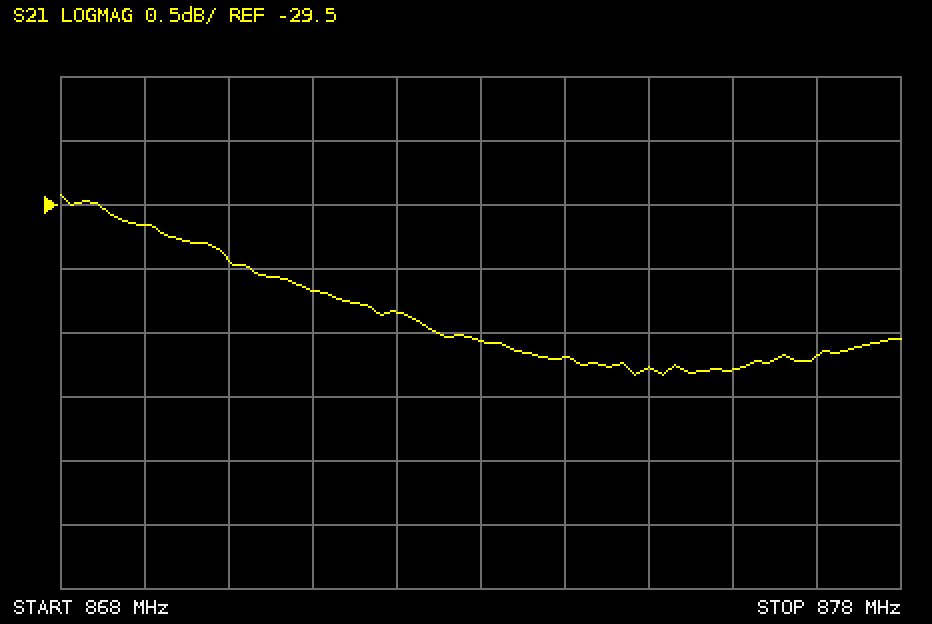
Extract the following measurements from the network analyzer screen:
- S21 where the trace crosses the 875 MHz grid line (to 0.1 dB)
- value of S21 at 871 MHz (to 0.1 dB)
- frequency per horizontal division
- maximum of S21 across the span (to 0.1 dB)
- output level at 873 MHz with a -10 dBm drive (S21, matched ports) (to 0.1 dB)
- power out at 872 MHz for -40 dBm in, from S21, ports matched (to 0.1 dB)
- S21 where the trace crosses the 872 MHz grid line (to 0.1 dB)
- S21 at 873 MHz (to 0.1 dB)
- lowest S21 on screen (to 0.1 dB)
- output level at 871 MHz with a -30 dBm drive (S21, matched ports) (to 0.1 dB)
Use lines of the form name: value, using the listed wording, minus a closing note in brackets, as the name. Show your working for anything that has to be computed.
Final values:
S21 where the trace crosses the 875 MHz grid line: -30.8 dB
value of S21 at 871 MHz: -30.2 dB
frequency per horizontal division: 1 MHz
maximum of S21 across the span: -29.4 dB
output level at 873 MHz with a -10 dBm drive (S21, matched ports): -10 dBm + (-30.6 dB) = -40.6 dBm
power out at 872 MHz for -40 dBm in, from S21, ports matched: -40 dBm + (-30.3 dB) = -70.3 dBm
S21 where the trace crosses the 872 MHz grid line: -30.3 dB
S21 at 873 MHz: -30.6 dB
lowest S21 on screen: -30.8 dB
output level at 871 MHz with a -30 dBm drive (S21, matched ports): -30 dBm + (-30.2 dB) = -60.2 dBm
